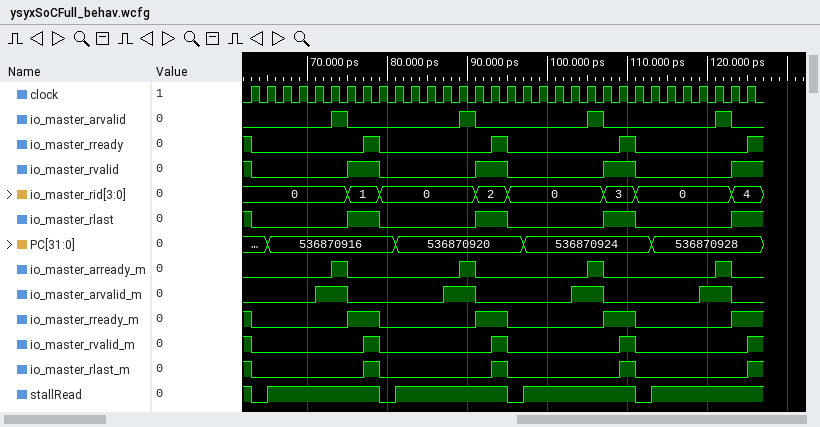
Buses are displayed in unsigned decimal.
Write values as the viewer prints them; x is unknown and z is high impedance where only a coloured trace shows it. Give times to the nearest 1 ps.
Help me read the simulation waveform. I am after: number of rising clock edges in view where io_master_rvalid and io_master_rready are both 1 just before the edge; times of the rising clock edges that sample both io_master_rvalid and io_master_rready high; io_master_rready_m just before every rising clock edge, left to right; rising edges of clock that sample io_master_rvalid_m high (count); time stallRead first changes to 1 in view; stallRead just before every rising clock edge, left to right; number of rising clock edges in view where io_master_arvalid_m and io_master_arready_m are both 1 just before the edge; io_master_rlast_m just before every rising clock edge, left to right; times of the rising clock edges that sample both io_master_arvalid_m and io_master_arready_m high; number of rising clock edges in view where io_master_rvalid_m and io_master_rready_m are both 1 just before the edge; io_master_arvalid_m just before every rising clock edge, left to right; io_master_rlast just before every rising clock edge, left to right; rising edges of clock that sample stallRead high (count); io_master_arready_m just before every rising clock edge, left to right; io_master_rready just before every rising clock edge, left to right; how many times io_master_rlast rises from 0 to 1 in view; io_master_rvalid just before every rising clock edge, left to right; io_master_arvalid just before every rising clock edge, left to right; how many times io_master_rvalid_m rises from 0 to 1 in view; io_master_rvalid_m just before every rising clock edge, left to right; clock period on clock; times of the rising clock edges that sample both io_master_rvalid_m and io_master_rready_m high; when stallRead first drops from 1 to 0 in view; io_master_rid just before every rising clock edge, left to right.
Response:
4
63 ps, 79 ps, 95 ps, 111 ps
1 0 0 0 0 0 0 1 1 0 0 0 0 0 0 1 1 0 0 0 0 0 0 1 1 0 0 0 0 0 0 1
4
65 ps
1 0 1 1 1 1 1 1 1 0 1 1 1 1 1 1 1 0 1 1 1 1 1 1 1 0 1 1 1 1 1 1
4
1 0 0 0 0 0 0 0 1 0 0 0 0 0 0 0 1 0 0 0 0 0 0 0 1 0 0 0 0 0 0 0
75 ps, 91 ps, 107 ps, 123 ps
4
0 0 0 0 0 1 1 0 0 0 0 0 0 1 1 0 0 0 0 0 0 1 1 0 0 0 0 0 0 1 1 0
1 0 0 0 0 0 0 1 1 0 0 0 0 0 0 1 1 0 0 0 0 0 0 1 1 0 0 0 0 0 0 1
28
0 0 0 0 0 0 1 0 0 0 0 0 0 0 1 0 0 0 0 0 0 0 1 0 0 0 0 0 0 0 1 0
1 0 0 0 0 0 0 0 1 0 0 0 0 0 0 0 1 0 0 0 0 0 0 0 1 0 0 0 0 0 0 0
4
1 0 0 0 0 0 0 1 1 0 0 0 0 0 0 1 1 0 0 0 0 0 0 1 1 0 0 0 0 0 0 1
0 0 0 0 0 0 1 0 0 0 0 0 0 0 1 0 0 0 0 0 0 0 1 0 0 0 0 0 0 0 1 0
4
1 0 0 0 0 0 0 0 1 0 0 0 0 0 0 0 1 0 0 0 0 0 0 0 1 0 0 0 0 0 0 0
2 ps
63 ps, 79 ps, 95 ps, 111 ps
63 ps
0, 0, 0, 0, 0, 0, 0, 1, 1, 0, 0, 0, 0, 0, 0, 2, 2, 0, 0, 0, 0, 0, 0, 3, 3, 0, 0, 0, 0, 0, 0, 4
